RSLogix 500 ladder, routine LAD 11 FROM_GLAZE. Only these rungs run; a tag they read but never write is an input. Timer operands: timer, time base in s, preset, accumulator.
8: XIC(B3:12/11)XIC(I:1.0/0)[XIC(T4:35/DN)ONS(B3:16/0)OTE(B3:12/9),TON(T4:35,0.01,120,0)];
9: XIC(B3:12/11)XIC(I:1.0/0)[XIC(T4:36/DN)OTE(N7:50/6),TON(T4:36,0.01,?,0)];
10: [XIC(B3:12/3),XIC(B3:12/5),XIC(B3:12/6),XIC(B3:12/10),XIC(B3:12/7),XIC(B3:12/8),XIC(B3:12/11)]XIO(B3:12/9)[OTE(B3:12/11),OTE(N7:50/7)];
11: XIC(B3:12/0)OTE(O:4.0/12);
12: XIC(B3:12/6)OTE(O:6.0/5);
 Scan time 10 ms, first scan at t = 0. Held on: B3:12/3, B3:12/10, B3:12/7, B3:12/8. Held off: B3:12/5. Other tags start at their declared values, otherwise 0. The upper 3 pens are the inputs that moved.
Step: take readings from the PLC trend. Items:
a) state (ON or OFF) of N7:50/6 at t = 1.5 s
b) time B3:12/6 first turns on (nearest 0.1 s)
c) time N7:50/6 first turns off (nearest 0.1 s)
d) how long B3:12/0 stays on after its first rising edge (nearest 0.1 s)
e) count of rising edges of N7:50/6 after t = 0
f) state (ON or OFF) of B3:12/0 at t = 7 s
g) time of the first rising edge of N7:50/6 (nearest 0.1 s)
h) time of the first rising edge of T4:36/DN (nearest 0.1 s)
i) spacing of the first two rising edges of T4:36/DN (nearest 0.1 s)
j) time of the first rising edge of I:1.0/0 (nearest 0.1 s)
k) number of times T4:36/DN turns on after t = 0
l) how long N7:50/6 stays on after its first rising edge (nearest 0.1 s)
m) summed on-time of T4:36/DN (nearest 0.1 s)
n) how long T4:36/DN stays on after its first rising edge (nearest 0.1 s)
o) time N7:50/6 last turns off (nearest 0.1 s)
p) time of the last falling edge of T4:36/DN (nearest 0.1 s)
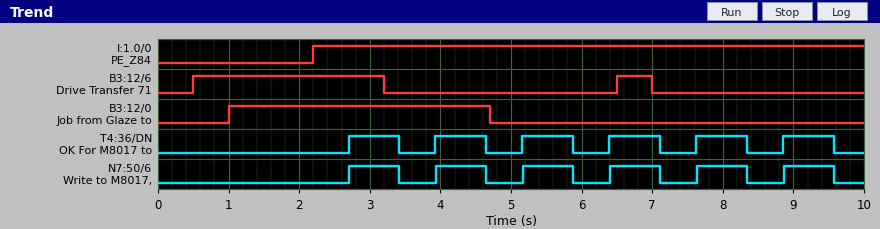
OFF
0.5 s
3.4 s
3.7 s
6
OFF
2.7 s
2.7 s
1.2 s
2.2 s
6
0.7 s
4.3 s
0.7 s
9.6 s
9.6 s
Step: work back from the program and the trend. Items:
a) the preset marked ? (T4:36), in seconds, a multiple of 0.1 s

0.5 s
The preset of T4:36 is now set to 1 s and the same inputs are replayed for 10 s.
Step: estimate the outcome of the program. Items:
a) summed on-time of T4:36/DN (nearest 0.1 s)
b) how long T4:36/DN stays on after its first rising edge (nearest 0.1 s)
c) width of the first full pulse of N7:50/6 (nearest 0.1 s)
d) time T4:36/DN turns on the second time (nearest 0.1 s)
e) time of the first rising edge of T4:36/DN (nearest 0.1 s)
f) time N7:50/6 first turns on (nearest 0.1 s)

1.3 s
0.2 s
0.2 s
4.4 s
3.2 s
3.2 s
